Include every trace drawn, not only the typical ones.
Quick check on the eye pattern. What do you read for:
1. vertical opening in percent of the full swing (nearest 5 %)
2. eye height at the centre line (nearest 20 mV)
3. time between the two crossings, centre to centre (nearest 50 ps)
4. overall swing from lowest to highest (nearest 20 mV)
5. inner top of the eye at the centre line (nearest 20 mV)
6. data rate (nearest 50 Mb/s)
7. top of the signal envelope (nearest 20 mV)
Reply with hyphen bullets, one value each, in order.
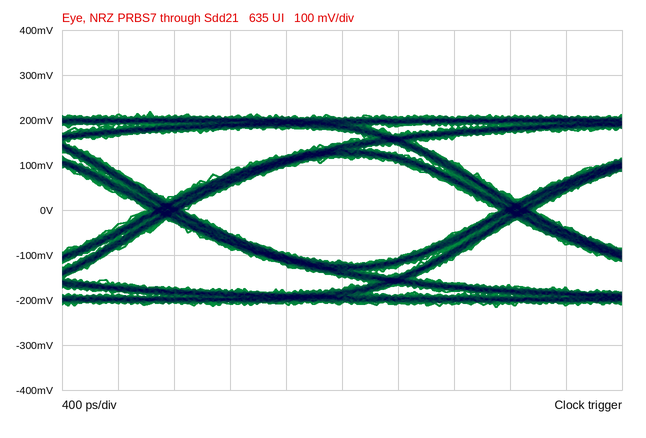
- 55 %
- 240 mV
- 2.50 ns
- 440 mV
- 120 mV
- 400 Mb/s
- 220 mV
